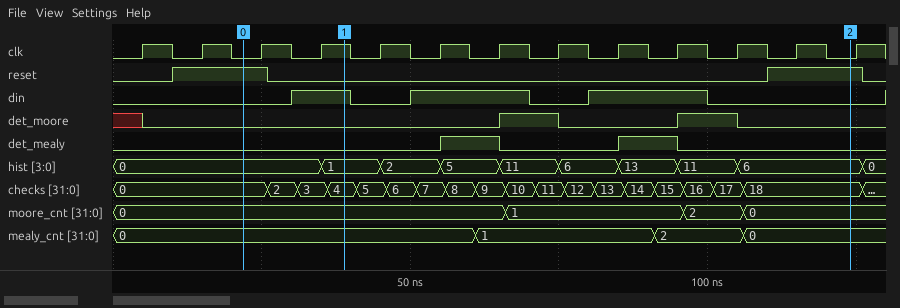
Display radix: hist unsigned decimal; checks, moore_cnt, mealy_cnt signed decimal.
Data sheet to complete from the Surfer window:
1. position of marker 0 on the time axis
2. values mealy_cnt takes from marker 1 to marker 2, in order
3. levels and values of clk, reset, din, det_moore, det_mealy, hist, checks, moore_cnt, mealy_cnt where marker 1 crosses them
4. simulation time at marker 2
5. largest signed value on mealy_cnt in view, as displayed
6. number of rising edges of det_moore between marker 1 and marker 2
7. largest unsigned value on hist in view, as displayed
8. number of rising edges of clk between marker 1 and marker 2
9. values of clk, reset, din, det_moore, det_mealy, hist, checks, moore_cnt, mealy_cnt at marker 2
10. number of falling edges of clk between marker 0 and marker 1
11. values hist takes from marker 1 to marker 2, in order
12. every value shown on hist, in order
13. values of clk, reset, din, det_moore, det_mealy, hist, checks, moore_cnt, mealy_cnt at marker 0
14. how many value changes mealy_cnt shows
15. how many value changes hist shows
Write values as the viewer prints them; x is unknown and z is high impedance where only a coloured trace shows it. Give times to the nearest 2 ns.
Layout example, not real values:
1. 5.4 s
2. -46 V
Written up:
1. 22 ns
2. 0, 1, 2, 0
3. clk=1, reset=0, din=1, det_moore=0, det_mealy=0, hist=1, checks=4, moore_cnt=0, mealy_cnt=0
4. 124 ns
5. 2
6. 2
7. 13
8. 8
9. clk=0, reset=1, din=0, det_moore=0, det_mealy=0, hist=6, checks=18, moore_cnt=0, mealy_cnt=0
10. 1
11. 1, 2, 5, 11, 6, 13, 11, 6
12. 0, 1, 2, 5, 11, 6, 13, 11, 6, 0
13. clk=0, reset=1, din=0, det_moore=0, det_mealy=0, hist=0, checks=0, moore_cnt=0, mealy_cnt=0
14. 3
15. 9
